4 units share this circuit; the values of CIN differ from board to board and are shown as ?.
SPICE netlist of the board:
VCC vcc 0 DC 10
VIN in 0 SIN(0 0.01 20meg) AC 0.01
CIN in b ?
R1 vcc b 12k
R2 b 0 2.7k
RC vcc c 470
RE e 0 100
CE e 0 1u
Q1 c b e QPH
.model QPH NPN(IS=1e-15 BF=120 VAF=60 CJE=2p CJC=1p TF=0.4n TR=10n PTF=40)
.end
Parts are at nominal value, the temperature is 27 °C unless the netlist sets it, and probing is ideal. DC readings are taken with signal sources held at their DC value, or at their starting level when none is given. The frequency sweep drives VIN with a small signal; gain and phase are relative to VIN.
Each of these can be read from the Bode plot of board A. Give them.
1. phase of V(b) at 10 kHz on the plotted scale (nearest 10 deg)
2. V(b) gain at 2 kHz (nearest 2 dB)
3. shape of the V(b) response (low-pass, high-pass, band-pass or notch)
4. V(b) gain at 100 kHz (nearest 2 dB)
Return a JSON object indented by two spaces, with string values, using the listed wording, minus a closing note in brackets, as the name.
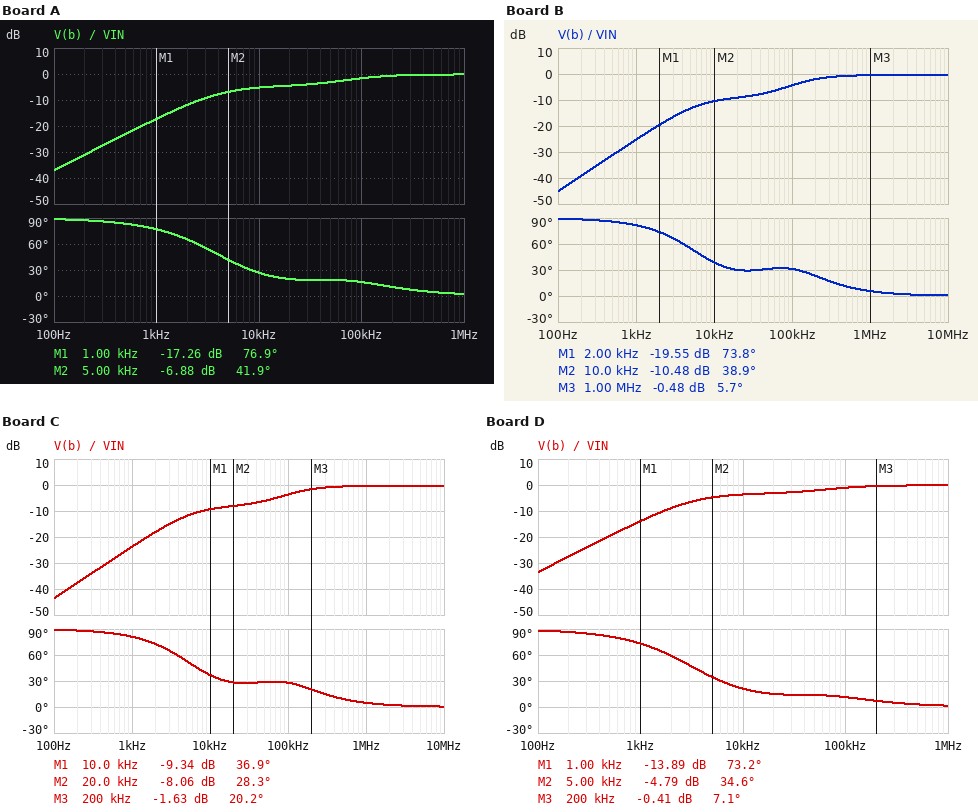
{
  "phase of V(b) at 10 kHz on the plotted scale": "30 deg",
  "V(b) gain at 2 kHz": "-12 dB",
  "shape of the V(b) response": "high-pass",
  "V(b) gain at 100 kHz": "-2 dB"
}
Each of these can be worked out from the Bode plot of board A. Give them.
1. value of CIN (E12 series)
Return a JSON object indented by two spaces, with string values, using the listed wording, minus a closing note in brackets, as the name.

{
  "value of CIN": "12 nF"
}
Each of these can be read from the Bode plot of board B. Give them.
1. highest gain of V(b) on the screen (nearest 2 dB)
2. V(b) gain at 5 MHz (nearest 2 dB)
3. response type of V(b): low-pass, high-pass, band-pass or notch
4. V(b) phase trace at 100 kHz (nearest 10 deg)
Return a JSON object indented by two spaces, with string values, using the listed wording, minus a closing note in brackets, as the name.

{
  "highest gain of V(b) on the screen": "0 dB",
  "V(b) gain at 5 MHz": "0 dB",
  "response type of V(b): low-pass, high-pass, band-pass or notch": "high-pass",
  "V(b) phase trace at 100 kHz": "30 deg"
}
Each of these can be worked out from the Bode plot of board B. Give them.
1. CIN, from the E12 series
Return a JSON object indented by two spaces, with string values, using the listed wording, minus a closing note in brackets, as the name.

{
  "CIN, from the E12 series": "4.7 nF"
}
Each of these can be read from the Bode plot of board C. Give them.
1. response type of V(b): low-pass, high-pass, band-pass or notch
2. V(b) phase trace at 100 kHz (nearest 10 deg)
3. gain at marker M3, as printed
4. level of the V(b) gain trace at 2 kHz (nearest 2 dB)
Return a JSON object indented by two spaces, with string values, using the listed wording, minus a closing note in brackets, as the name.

{
  "response type of V(b): low-pass, high-pass, band-pass or notch": "high-pass",
  "V(b) phase trace at 100 kHz": "30 deg",
  "gain at marker M3, as printed": "-1.63 dB",
  "level of the V(b) gain trace at 2 kHz": "-18 dB"
}
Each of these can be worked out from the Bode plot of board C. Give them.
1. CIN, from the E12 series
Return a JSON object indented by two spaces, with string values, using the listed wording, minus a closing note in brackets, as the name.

{
  "CIN, from the E12 series": "5.6 nF"
}
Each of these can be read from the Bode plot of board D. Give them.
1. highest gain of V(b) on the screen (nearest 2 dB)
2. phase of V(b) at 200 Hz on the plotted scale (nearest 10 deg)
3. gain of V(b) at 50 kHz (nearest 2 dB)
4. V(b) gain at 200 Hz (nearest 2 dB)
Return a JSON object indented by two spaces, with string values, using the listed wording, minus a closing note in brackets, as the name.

{
  "highest gain of V(b) on the screen": "0 dB",
  "phase of V(b) at 200 Hz on the plotted scale": "90 deg",
  "gain of V(b) at 50 kHz": "-2 dB",
  "V(b) gain at 200 Hz": "-28 dB"
}
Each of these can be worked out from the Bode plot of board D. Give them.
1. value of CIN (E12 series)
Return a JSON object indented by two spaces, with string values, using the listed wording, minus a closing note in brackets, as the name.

{
  "value of CIN": "18 nF"
}
